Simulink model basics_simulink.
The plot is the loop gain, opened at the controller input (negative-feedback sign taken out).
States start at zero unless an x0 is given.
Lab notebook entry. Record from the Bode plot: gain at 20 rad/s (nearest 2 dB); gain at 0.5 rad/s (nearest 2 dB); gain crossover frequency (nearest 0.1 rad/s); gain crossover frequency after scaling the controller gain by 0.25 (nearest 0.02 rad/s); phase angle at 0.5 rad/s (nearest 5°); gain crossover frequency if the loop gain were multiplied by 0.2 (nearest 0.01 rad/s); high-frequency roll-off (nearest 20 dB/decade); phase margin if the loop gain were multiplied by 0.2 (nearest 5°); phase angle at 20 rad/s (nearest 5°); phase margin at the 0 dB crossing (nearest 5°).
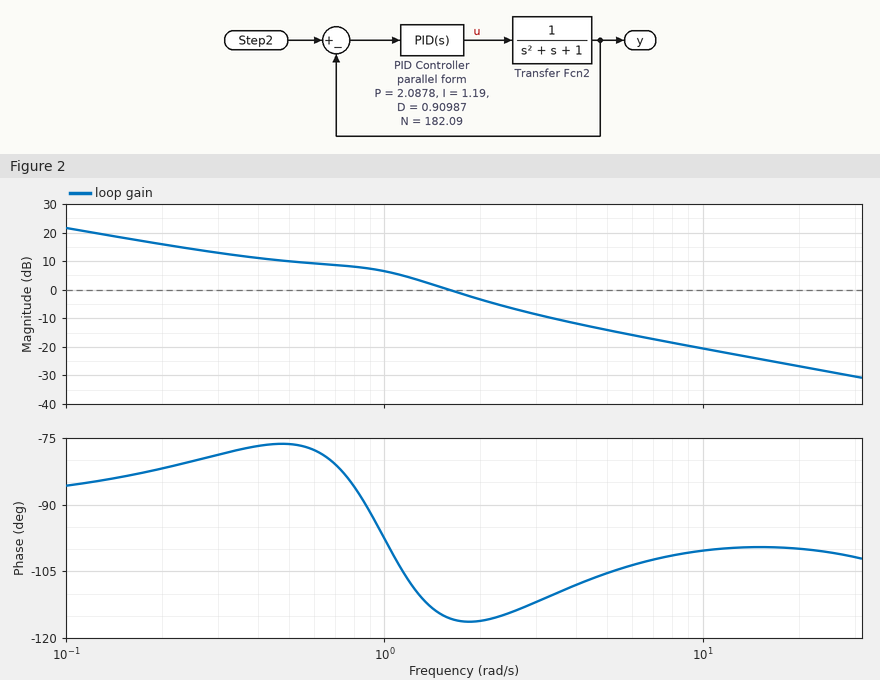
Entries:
-26 dB
10 dB
1.6 rad/s
0.34 rad/s
-75°
0.26 rad/s
-20 dB/decade
100°
-100°
65°
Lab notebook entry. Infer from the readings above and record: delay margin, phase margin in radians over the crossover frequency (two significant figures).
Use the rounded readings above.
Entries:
0.71 s
